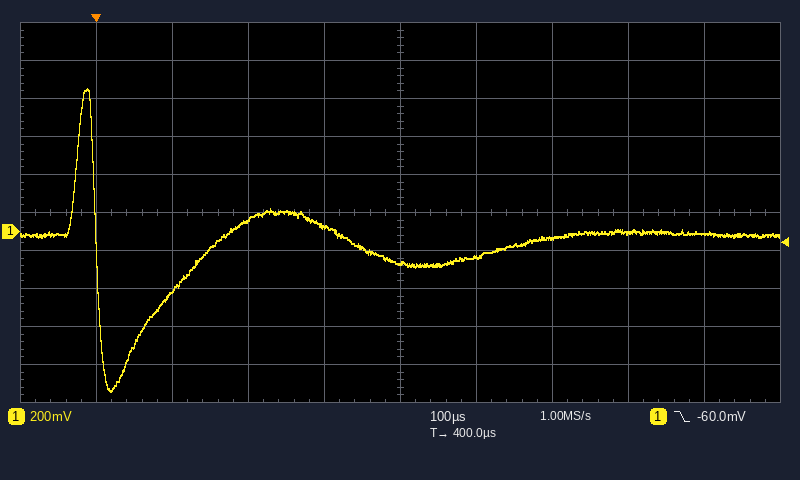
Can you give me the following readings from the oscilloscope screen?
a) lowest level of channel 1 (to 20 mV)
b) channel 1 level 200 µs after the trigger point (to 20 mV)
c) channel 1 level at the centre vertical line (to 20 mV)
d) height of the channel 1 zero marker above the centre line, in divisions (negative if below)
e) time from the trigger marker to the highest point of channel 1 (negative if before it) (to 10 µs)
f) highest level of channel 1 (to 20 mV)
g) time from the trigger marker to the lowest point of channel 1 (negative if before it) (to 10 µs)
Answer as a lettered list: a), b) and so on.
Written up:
a) -840 mV
b) 60 mV
c) -160 mV
d) -0.5 div
e) -10 µs
f) 760 mV
g) +20 µs
